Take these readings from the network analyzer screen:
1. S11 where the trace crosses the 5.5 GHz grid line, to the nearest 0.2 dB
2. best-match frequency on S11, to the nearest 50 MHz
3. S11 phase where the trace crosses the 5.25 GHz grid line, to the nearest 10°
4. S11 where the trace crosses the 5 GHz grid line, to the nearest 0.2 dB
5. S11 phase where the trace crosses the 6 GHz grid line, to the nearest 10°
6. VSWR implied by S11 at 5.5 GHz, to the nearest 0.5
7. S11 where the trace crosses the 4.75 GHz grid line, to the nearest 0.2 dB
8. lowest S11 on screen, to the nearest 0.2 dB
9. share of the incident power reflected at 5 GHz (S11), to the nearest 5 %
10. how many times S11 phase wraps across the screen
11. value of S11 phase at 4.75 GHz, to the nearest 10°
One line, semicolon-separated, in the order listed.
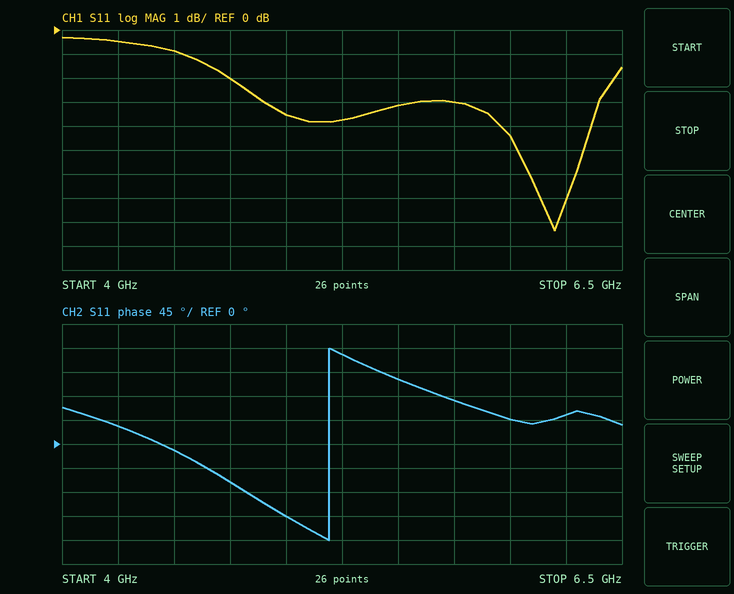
-3.2 dB; 6.20 GHz; 170°; -3.6 dB; 50°; 5.5; -2.0 dB; -8.4 dB; 45 %; 1; -70°
